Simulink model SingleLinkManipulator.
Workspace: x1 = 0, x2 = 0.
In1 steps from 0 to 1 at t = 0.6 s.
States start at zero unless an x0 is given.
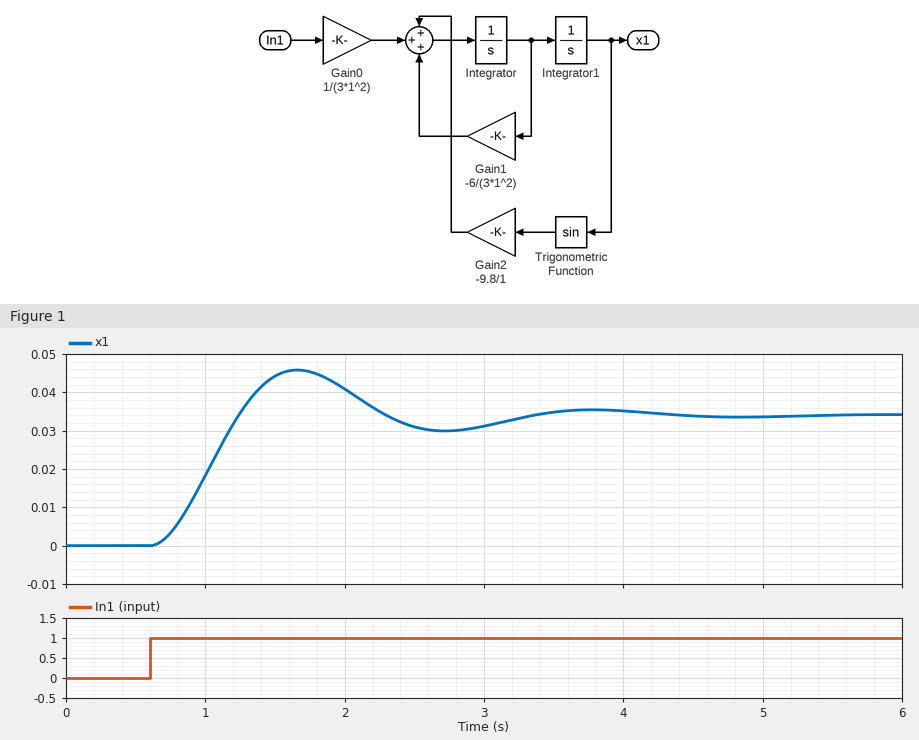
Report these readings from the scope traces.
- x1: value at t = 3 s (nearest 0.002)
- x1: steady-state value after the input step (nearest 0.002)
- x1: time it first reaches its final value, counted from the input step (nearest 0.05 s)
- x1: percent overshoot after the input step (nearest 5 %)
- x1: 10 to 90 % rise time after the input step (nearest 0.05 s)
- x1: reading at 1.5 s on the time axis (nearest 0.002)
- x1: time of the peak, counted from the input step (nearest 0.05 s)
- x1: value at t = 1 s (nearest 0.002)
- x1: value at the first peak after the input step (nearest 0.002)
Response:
0.032
0.034
0.65 s
35 %
0.45 s
0.044
1.05 s
0.018
0.046
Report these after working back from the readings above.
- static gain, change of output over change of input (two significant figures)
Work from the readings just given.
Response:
0.034
